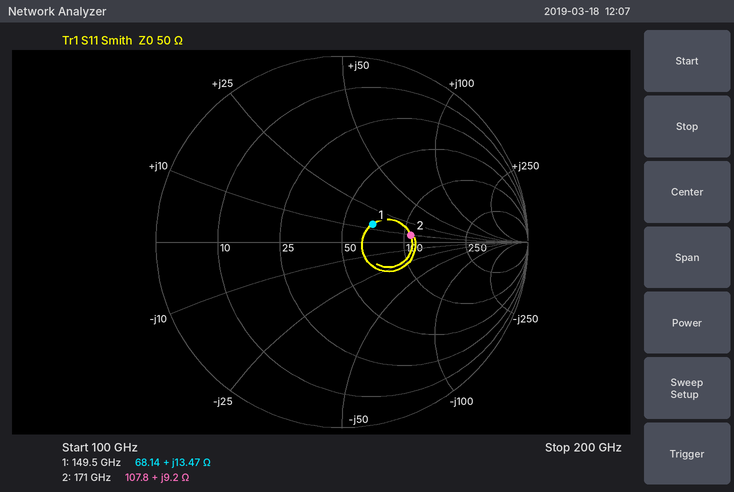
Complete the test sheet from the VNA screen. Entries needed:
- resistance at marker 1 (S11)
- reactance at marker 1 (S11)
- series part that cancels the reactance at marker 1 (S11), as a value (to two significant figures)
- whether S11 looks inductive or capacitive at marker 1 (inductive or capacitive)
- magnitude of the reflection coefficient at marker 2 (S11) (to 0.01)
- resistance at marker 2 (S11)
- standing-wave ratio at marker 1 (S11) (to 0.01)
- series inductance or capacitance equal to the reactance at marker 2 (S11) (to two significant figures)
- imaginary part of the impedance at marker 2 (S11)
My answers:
68.14 Ω
+13.47 Ω
79 fF
inductive
0.37
107.8 Ω
1.47
8.6 pH
+9.2 Ω
